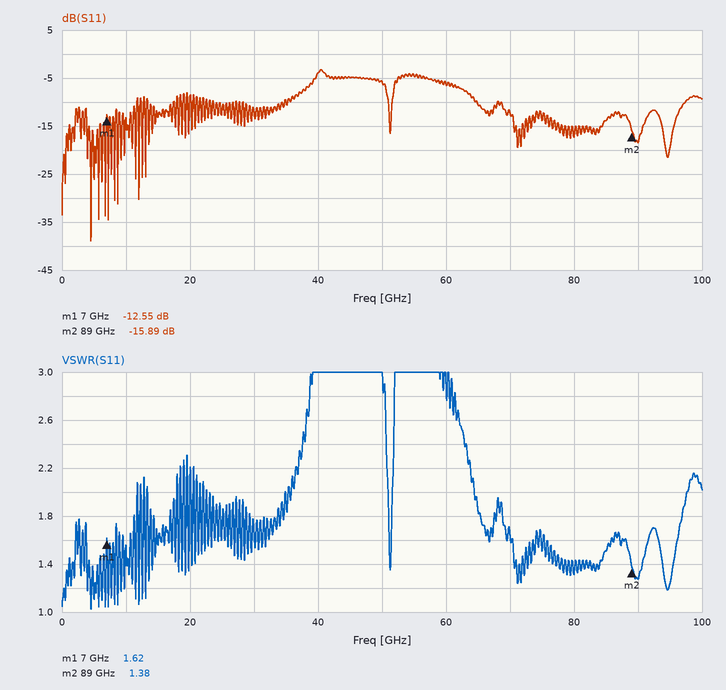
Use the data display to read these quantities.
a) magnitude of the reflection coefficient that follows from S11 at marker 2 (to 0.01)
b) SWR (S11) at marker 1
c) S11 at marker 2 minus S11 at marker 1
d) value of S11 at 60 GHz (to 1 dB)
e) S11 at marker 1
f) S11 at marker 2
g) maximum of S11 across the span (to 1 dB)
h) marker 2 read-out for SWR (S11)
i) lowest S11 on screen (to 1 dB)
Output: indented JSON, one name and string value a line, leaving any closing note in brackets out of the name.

{
  "magnitude of the reflection coefficient that follows from S11 at marker 2": "0.16",
  "SWR (S11) at marker 1": "1.62",
  "S11 at marker 2 minus S11 at marker 1": "-3.34 dB",
  "value of S11 at 60 GHz": "-6 dB",
  "S11 at marker 1": "-12.55 dB",
  "S11 at marker 2": "-15.89 dB",
  "maximum of S11 across the span": "-3 dB",
  "marker 2 read-out for SWR": "1.38",
  "lowest S11 on screen": "-39 dB"
}
